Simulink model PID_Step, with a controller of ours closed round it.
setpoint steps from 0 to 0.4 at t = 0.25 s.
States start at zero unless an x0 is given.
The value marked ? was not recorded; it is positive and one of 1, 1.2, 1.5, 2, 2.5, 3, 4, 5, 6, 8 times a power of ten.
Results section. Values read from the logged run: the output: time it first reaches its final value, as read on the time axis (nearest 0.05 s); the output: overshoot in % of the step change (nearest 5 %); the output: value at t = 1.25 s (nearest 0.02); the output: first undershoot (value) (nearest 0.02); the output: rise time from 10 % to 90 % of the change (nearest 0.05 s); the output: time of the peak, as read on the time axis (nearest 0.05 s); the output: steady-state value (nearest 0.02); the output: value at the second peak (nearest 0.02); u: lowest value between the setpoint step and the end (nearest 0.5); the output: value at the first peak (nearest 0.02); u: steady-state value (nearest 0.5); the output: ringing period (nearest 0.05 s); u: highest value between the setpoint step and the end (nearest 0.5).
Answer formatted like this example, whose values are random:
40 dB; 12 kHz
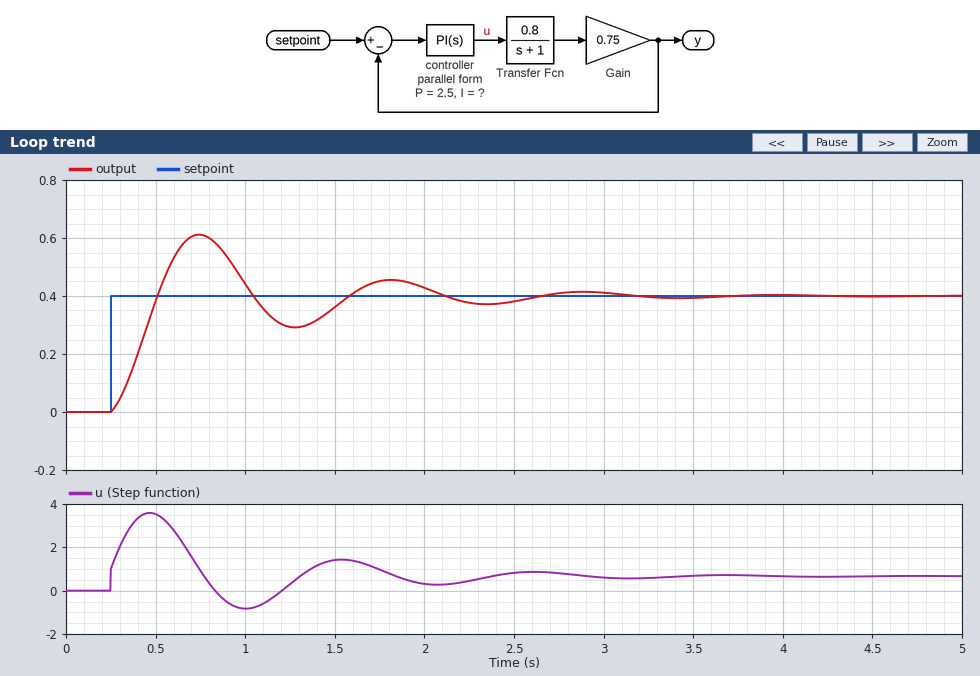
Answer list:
0.50 s; 55 %; 0.30; 0.30; 0.20 s; 0.75 s; 0.40; 0.46; -1.0; 0.62; 0.5; 1.05 s; 3.5
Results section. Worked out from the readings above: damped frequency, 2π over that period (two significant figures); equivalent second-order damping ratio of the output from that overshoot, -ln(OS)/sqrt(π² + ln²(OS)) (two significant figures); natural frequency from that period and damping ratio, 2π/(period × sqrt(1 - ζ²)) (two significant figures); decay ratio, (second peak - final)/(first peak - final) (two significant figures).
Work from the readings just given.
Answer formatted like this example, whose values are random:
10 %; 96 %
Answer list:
6.0 rad/s; 0.19; 6.1 rad/s; 0.27
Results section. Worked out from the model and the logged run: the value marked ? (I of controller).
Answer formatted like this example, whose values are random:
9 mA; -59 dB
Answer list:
60
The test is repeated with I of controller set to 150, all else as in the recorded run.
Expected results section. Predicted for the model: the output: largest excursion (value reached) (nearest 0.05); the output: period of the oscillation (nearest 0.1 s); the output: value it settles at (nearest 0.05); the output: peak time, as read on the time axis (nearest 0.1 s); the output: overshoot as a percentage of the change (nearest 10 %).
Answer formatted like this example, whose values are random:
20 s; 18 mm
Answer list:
0.65; 0.7 s; 0.40; 0.6 s; 70 %
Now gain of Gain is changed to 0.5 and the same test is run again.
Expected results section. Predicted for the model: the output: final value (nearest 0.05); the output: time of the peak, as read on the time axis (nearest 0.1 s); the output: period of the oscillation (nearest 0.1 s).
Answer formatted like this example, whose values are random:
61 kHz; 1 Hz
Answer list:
0.40; 0.9 s; 1.3 s
